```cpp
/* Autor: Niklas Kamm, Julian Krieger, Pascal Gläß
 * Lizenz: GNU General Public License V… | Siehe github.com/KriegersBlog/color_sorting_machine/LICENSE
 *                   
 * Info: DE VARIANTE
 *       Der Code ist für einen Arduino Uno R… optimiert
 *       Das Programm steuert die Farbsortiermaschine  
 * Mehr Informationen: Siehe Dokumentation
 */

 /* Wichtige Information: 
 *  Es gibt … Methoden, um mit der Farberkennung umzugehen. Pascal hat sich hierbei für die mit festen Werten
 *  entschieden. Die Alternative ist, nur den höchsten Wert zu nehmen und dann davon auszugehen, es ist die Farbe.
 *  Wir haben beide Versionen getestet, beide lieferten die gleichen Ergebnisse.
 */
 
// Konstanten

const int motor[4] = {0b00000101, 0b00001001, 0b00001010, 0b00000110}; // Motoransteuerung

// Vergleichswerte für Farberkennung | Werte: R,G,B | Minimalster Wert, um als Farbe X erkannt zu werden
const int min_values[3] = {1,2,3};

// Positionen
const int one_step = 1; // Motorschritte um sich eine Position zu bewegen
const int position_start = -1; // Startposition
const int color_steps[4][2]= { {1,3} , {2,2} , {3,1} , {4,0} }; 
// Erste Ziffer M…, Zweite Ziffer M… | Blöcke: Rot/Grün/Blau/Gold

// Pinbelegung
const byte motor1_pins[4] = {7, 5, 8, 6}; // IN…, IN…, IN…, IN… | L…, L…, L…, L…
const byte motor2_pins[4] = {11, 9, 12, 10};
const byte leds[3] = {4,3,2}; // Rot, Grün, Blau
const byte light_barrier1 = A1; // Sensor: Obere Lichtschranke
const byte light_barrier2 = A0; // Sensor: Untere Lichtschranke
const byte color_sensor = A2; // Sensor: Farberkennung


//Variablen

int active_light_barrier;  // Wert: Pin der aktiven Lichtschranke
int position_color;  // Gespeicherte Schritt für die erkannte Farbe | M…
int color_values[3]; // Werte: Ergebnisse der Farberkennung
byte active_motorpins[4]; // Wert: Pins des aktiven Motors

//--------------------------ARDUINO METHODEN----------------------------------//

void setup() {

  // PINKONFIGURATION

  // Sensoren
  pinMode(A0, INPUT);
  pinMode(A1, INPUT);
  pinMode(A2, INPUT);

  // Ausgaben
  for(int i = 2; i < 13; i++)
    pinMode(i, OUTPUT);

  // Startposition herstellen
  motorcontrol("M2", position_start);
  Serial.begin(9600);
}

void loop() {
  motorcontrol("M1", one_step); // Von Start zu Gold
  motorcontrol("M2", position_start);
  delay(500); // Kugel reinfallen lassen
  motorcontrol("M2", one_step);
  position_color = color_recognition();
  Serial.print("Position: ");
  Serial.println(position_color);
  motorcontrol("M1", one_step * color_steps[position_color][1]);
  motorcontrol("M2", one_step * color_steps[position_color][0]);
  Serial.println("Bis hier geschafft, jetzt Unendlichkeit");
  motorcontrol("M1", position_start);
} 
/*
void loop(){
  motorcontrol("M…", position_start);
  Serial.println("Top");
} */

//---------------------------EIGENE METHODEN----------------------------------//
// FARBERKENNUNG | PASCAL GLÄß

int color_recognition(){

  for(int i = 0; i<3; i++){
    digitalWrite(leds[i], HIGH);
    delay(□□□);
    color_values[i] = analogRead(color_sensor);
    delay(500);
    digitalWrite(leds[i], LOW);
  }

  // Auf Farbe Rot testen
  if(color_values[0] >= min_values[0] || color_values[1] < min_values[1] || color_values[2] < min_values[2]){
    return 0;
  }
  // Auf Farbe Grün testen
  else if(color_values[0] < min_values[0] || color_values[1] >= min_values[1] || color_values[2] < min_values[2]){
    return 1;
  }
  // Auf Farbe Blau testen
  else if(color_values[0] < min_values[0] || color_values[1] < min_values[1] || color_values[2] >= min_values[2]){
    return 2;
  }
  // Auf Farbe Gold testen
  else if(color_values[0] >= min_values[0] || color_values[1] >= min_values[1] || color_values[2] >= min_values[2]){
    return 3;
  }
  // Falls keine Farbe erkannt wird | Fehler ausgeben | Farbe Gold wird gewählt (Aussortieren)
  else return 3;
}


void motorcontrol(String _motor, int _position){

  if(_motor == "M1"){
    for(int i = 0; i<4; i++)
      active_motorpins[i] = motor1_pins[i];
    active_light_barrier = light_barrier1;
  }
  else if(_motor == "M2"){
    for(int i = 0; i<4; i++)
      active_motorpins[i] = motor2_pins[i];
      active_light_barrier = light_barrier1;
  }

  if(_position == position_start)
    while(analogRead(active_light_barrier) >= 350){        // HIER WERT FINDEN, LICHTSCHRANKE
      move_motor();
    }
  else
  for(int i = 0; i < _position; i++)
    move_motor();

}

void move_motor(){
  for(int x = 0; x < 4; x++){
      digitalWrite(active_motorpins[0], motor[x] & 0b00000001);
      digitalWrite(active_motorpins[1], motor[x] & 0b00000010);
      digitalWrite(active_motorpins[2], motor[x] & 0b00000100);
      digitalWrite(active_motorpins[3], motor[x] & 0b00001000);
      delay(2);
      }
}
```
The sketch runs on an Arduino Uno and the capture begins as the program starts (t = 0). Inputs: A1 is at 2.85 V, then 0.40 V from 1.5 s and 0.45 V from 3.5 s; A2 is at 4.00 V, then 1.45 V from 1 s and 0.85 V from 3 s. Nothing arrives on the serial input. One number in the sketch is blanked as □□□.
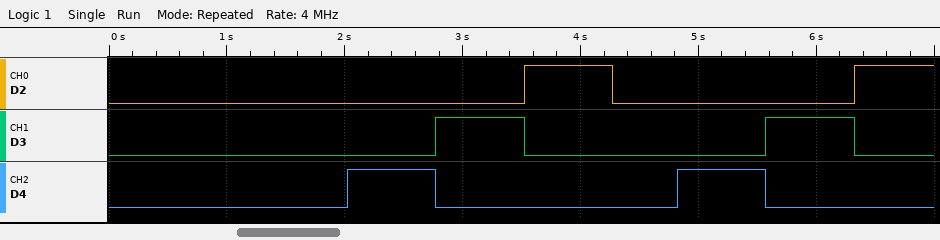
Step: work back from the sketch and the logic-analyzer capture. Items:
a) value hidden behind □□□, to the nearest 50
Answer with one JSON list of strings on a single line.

["250"]
